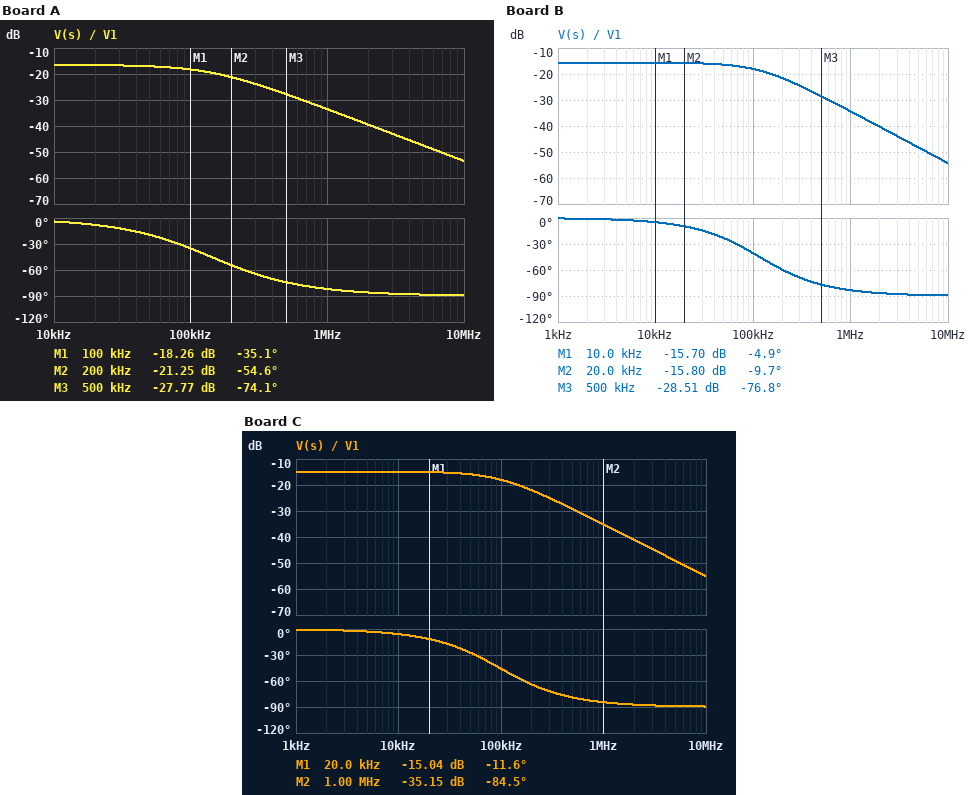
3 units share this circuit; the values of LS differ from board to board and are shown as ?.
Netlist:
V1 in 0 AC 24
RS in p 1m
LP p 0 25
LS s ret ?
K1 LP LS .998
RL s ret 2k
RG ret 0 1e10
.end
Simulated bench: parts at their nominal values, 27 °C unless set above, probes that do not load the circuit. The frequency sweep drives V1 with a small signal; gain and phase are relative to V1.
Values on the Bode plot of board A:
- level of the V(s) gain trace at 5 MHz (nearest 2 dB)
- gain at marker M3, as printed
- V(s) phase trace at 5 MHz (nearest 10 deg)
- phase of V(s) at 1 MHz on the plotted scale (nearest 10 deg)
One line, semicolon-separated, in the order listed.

-48 dB; -27.77 dB; -90 deg; -80 deg
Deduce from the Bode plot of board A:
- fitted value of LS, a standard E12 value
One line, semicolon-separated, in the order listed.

560 mH
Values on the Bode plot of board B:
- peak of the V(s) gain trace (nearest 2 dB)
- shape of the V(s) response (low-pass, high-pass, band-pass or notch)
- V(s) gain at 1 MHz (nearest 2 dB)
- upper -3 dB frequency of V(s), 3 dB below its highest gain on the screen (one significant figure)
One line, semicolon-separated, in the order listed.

-16 dB; low-pass; -34 dB; 100 kHz
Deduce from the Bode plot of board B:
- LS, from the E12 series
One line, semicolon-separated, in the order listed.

680 mH
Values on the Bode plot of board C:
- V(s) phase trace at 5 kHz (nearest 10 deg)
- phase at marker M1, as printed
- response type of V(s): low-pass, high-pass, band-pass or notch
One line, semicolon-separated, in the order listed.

0 deg; -11.6 deg; low-pass
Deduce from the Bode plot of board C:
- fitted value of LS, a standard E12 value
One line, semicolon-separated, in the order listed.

820 mH
